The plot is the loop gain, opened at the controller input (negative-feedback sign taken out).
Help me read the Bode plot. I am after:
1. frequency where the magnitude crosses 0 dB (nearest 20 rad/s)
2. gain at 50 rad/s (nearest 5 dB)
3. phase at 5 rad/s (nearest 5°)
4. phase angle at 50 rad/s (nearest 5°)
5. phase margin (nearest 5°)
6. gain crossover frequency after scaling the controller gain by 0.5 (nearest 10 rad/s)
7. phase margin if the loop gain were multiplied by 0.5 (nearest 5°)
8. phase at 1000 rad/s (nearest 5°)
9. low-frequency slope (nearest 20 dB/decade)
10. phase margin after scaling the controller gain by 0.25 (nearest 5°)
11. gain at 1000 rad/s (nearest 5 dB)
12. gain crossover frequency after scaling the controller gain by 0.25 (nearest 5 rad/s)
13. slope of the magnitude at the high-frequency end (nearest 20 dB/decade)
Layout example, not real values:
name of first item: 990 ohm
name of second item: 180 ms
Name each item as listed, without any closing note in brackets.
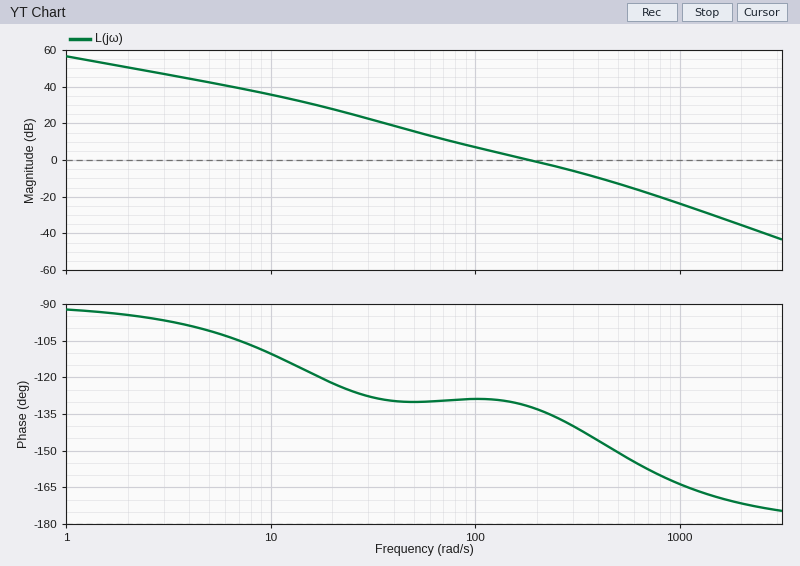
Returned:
frequency where the magnitude crosses 0 dB: 180 rad/s
gain at 50 rad/s: 15 dB
phase at 5 rad/s: -100°
phase angle at 50 rad/s: -130°
phase margin: 50°
gain crossover frequency after scaling the controller gain by 0.5: 110 rad/s
phase margin if the loop gain were multiplied by 0.5: 50°
phase at 1000 rad/s: -165°
low-frequency slope: -20 dB/decade
phase margin after scaling the controller gain by 0.25: 50°
gain at 1000 rad/s: -25 dB
gain crossover frequency after scaling the controller gain by 0.25: 65 rad/s
slope of the magnitude at the high-frequency end: -40 dB/decade
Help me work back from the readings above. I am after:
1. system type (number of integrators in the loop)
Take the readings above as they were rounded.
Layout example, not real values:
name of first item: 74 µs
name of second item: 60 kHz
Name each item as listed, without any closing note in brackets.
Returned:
system type: 1
